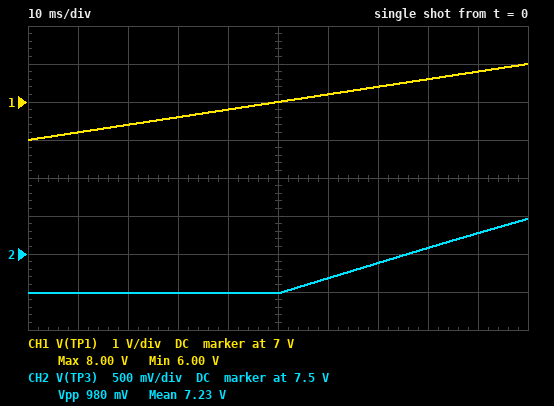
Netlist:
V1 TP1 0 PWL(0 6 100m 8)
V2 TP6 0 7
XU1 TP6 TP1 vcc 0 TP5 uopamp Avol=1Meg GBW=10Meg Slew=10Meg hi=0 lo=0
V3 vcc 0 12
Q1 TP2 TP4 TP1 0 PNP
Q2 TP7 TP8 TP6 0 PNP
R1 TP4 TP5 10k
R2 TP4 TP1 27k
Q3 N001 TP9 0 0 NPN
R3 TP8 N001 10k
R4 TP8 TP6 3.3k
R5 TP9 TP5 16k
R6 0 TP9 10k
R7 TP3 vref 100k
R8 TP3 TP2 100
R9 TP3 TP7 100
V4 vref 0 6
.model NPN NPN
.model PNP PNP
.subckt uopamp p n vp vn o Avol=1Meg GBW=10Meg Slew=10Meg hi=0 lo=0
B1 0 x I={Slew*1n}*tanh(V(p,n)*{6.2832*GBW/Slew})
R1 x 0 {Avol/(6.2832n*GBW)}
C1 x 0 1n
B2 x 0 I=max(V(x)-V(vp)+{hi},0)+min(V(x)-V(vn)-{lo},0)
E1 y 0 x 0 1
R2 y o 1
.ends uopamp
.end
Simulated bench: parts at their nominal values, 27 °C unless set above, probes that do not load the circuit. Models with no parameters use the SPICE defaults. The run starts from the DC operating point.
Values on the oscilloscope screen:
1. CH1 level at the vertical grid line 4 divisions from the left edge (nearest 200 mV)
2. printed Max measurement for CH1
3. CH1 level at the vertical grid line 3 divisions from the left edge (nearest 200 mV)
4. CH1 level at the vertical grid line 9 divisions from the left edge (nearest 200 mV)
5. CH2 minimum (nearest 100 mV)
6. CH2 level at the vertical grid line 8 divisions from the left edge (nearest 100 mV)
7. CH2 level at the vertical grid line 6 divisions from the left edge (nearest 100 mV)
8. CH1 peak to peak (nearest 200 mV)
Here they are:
6.8 V
8.00 V
6.6 V
7.8 V
7.0 V
7.6 V
7.2 V
2.0 V
